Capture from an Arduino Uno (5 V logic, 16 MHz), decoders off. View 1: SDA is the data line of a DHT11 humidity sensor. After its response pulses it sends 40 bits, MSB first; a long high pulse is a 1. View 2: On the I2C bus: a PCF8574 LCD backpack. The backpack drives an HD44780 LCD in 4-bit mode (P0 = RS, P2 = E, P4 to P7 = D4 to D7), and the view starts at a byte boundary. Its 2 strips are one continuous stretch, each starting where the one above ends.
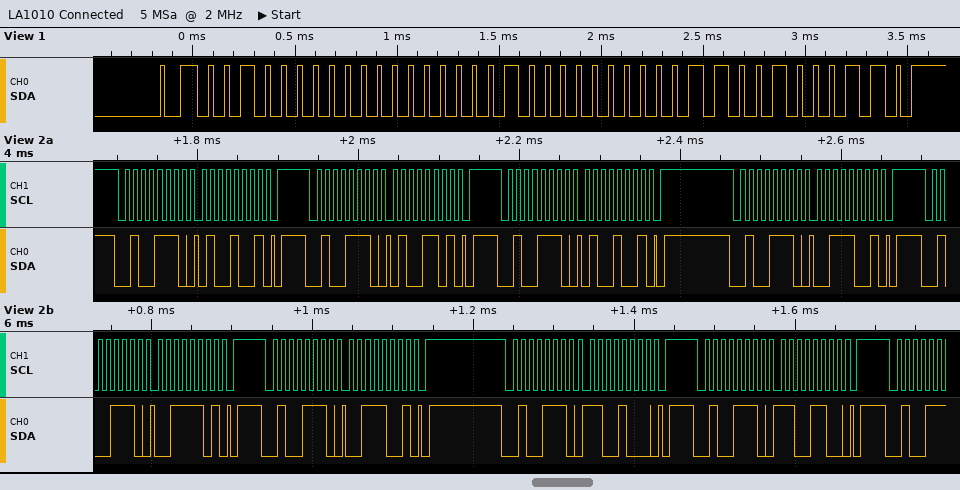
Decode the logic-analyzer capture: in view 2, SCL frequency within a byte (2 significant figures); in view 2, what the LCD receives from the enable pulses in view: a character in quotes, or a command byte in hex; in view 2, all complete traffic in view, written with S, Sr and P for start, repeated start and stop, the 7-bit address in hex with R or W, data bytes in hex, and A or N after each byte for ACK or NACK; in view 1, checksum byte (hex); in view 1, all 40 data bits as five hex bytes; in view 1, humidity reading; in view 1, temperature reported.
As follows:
100 kHz
'C'
S 27W A 49 A P S 27W A 4D A P S 27W A 49 A P S 27W A 39 A P S 27W A 3D A P S 27W A 39 A P S 27W A C8 A P S 27W A CC A P
0x46
20 00 20 06 46
32 %
32.6 °C
